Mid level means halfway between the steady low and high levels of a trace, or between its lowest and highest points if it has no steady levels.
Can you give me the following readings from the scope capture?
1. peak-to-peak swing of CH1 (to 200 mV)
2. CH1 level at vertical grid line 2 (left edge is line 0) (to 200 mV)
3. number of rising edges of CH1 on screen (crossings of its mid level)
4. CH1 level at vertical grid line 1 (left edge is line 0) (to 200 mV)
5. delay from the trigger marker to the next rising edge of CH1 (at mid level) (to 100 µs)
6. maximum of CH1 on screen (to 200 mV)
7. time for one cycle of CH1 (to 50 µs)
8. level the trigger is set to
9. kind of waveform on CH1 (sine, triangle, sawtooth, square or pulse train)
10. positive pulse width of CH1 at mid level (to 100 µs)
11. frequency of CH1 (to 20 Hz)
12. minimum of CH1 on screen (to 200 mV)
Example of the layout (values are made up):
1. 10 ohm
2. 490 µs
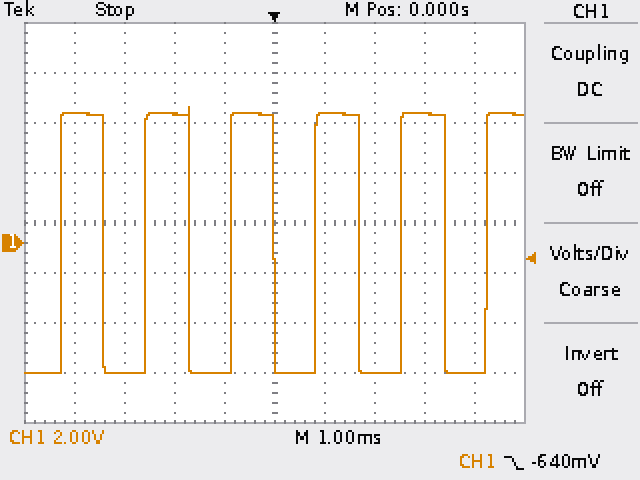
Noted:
1. 10.6 V
2. -5.2 V
3. 6
4. 5.2 V
5. 800 µs
6. 5.4 V
7. 1.70 ms
8. -640 mV
9. square
10. 900 µs
11. 580 Hz
12. -5.2 V
